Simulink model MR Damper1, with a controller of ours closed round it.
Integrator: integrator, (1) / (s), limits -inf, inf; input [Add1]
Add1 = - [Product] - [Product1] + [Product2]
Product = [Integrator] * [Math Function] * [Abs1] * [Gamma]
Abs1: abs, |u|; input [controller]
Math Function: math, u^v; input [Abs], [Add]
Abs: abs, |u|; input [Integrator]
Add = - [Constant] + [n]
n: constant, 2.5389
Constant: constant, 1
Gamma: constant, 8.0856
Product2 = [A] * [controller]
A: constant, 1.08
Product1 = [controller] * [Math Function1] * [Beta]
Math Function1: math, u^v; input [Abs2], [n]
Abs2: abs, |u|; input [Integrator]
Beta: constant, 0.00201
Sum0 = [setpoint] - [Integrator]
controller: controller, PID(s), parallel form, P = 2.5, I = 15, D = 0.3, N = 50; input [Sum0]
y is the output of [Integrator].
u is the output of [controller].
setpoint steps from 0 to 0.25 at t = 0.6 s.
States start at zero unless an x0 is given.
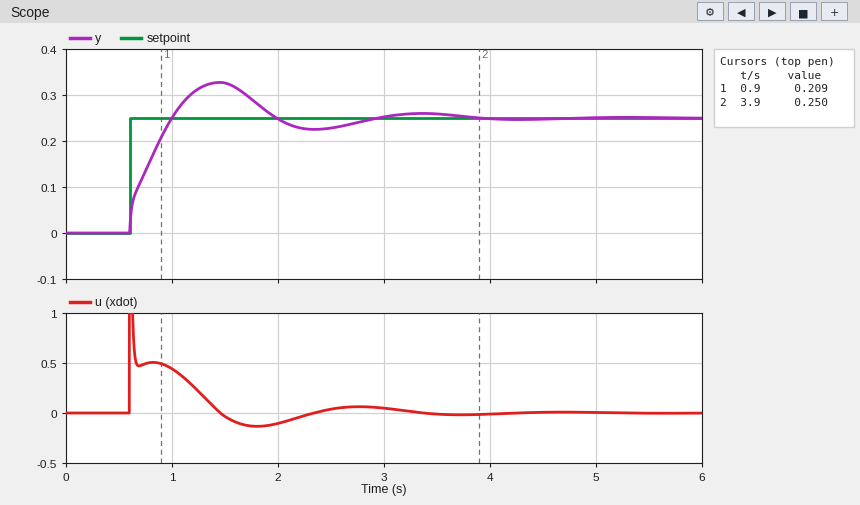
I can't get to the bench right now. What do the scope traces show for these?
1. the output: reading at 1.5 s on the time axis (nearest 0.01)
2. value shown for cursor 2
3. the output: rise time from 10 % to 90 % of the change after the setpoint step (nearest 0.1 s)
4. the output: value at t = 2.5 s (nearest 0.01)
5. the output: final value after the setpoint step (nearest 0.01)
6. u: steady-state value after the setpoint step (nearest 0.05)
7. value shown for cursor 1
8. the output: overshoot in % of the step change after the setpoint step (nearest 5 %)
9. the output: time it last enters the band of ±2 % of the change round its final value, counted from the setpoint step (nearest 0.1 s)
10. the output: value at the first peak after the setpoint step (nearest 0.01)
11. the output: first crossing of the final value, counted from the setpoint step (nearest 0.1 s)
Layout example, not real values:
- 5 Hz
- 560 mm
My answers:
- 0.33
- 0.250
- 0.3 s
- 0.23
- 0.25
- 0.00
- 0.209
- 30 %
- 3.1 s
- 0.33
- 0.4 s
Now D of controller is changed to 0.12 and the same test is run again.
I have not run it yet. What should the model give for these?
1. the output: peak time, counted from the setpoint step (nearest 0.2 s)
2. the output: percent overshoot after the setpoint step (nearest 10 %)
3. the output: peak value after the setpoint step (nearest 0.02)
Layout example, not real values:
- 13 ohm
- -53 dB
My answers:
- 0.8 s
- 30 %
- 0.34
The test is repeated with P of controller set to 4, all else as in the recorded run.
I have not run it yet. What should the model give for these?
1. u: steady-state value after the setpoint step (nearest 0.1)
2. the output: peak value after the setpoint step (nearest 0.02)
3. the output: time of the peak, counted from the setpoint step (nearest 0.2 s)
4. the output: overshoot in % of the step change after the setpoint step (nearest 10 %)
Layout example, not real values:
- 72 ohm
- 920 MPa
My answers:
- 0.0
- 0.30
- 0.8 s
- 20 %
